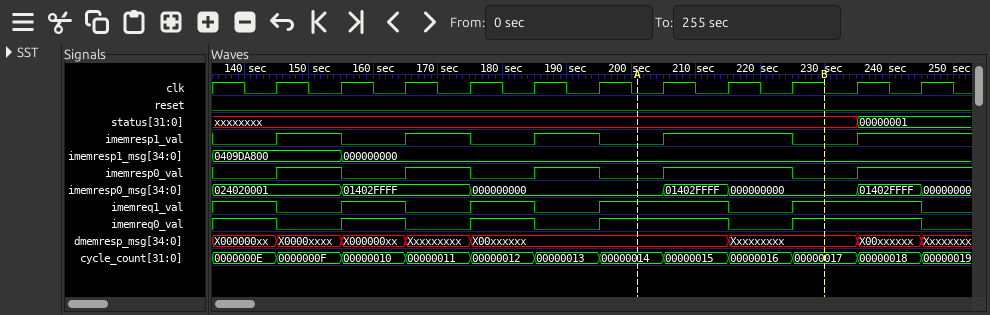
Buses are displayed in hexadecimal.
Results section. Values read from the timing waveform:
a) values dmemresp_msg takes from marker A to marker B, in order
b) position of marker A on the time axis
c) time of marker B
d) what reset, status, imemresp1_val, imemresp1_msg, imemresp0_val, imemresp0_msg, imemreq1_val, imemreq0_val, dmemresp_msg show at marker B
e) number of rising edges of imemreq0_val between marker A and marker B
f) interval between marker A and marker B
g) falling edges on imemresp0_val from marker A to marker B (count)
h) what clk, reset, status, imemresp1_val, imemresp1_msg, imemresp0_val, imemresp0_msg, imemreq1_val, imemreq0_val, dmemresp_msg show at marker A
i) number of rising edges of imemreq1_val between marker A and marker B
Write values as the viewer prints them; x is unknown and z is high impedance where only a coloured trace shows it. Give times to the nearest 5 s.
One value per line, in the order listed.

X00xxxxxx, Xxxxxxxxx
200 s
230 s
reset=0, status=xxxxxxxx, imemresp1_val=0, imemresp1_msg=000000000, imemresp0_val=0, imemresp0_msg=000000000, imemreq1_val=1, imemreq0_val=1, dmemresp_msg=Xxxxxxxxx
1
30 s
1
clk=0, reset=0, status=xxxxxxxx, imemresp1_val=0, imemresp1_msg=000000000, imemresp0_val=0, imemresp0_msg=000000000, imemreq1_val=1, imemreq0_val=1, dmemresp_msg=X00xxxxxx
1
